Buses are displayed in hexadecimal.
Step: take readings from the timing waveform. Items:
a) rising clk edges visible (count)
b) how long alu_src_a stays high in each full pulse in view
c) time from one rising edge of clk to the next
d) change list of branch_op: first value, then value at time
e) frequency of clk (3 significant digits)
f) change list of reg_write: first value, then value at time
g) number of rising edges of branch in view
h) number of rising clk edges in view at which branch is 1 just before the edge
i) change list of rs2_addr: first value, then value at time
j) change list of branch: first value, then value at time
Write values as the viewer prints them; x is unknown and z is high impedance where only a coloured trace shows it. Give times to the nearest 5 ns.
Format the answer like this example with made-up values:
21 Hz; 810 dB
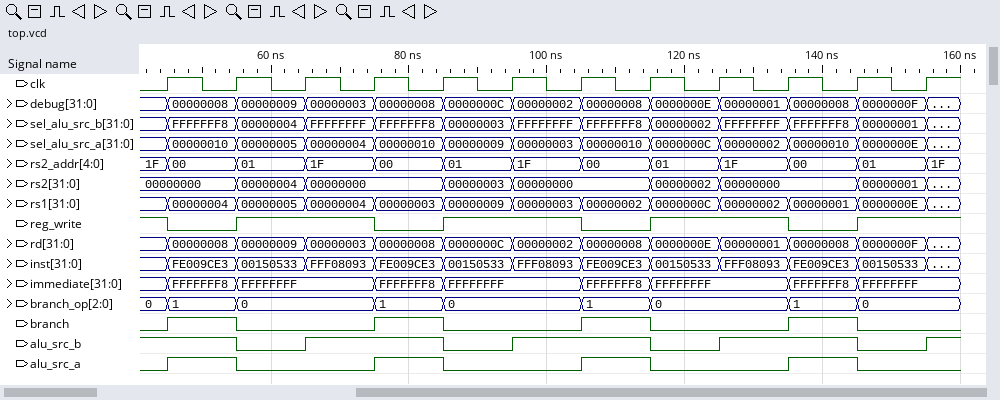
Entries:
12; 10 ns, 10 ns, 10 ns, 10 ns; 10 ns; 0, 1 at 45 ns, 0 at 55 ns, 1 at 75 ns, 0 at 85 ns, 1 at 105 ns, 0 at 115 ns, 1 at 135 ns, 0 at 145 ns; 100 MHz; 1, 0 at 45 ns, 1 at 55 ns, 0 at 75 ns, 1 at 85 ns, 0 at 105 ns, 1 at 115 ns, 0 at 135 ns, 1 at 145 ns; 4; 4; 1F, 00 at 45 ns, 01 at 55 ns, 1F at 65 ns, 00 at 75 ns, 01 at 85 ns, 1F at 95 ns, 00 at 105 ns, 01 at 115 ns, 1F at 125 ns, 00 at 135 ns, 01 at 145 ns, 1F at 155 ns; 0, 1 at 45 ns, 0 at 55 ns, 1 at 75 ns, 0 at 85 ns, 1 at 105 ns, 0 at 115 ns, 1 at 135 ns, 0 at 145 ns
